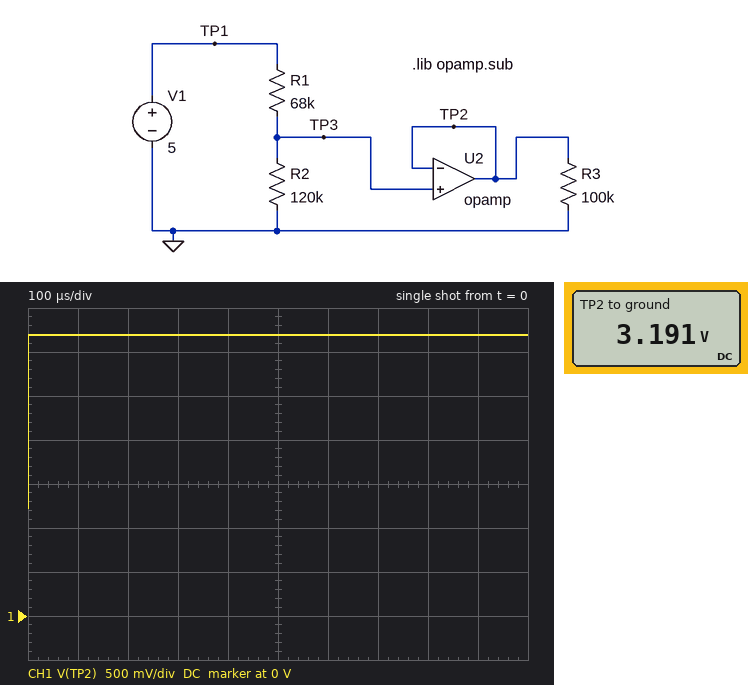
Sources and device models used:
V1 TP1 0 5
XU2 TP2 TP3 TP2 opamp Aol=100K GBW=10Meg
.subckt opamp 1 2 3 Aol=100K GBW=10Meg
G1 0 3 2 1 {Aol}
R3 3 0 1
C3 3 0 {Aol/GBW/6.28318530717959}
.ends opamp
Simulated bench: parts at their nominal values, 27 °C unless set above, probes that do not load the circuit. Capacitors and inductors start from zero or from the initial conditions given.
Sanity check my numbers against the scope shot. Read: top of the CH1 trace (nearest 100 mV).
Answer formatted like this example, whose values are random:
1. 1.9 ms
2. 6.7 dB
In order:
1. 3.2 V
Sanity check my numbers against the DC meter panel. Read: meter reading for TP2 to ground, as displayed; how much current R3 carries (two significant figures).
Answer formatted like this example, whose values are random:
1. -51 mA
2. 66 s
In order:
1. 3.191 V
2. 32 µA
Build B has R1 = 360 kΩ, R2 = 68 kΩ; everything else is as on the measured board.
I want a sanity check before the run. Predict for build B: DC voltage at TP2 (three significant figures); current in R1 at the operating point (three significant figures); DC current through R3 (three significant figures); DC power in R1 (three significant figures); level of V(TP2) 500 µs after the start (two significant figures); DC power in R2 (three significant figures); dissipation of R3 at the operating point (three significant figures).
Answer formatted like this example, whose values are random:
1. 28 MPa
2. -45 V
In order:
1. 794 mV
2. 11.7 µA
3. 7.94 µA
4. 49.1 µW
5. 790 mV
6. 9.28 µW
7. 6.31 µW
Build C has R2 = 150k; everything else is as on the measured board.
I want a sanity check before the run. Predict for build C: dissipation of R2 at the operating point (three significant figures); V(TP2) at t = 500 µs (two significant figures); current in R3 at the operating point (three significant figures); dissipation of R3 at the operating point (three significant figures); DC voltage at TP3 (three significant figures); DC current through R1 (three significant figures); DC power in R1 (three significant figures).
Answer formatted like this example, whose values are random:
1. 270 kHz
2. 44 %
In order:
1. 78.9 µW
2. 3.4 V
3. 34.4 µA
4. 118 µW
5. 3.44 V
6. 22.9 µA
7. 35.8 µW
